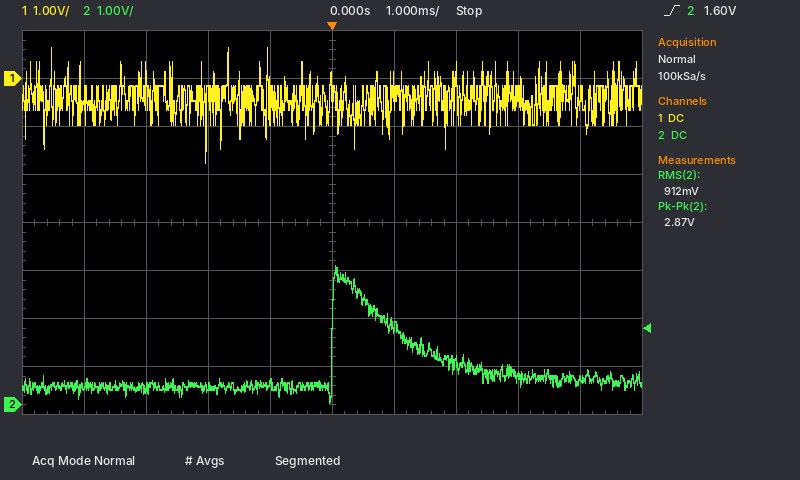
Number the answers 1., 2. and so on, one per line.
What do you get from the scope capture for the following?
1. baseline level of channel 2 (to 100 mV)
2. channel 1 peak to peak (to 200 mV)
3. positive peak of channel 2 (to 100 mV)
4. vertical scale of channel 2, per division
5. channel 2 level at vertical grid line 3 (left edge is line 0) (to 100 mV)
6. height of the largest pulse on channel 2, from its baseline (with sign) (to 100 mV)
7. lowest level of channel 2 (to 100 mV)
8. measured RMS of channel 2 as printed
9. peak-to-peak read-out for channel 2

1. 400 mV
2. 2.4 V
3. 2.9 V
4. 1 V
5. 400 mV
6. +2.5 V
7. 0.0 V
8. 912 mV
9. 2.87 V
